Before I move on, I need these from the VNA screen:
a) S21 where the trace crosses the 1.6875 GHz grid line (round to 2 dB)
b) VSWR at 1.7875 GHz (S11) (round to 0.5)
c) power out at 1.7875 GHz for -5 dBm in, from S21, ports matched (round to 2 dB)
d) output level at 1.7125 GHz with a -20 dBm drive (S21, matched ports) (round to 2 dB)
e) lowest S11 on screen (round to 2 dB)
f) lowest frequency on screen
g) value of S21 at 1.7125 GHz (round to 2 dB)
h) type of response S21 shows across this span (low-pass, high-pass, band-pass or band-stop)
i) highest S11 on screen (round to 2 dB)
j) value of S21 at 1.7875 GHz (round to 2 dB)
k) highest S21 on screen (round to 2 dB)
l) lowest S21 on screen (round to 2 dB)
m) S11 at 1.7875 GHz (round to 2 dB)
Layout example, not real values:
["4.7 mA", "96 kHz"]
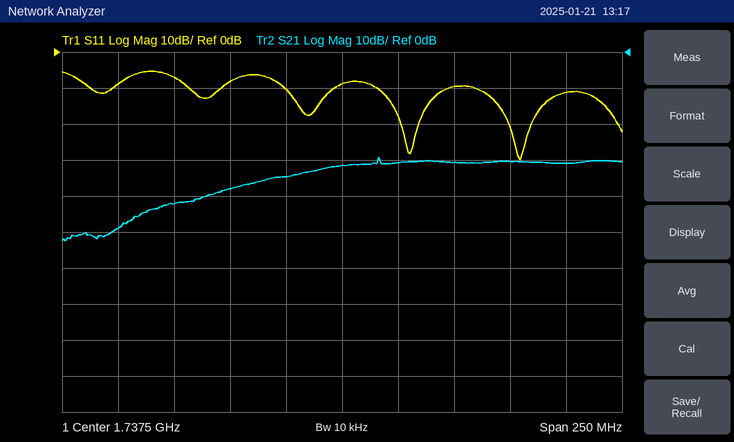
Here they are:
["-38 dB", "2.0", "-36 dBm", "-54 dBm", "-30 dB", "1.6125 GHz", "-34 dB", "high-pass", "-6 dB", "-30 dB", "-30 dB", "-52 dB", "-10 dB"]
